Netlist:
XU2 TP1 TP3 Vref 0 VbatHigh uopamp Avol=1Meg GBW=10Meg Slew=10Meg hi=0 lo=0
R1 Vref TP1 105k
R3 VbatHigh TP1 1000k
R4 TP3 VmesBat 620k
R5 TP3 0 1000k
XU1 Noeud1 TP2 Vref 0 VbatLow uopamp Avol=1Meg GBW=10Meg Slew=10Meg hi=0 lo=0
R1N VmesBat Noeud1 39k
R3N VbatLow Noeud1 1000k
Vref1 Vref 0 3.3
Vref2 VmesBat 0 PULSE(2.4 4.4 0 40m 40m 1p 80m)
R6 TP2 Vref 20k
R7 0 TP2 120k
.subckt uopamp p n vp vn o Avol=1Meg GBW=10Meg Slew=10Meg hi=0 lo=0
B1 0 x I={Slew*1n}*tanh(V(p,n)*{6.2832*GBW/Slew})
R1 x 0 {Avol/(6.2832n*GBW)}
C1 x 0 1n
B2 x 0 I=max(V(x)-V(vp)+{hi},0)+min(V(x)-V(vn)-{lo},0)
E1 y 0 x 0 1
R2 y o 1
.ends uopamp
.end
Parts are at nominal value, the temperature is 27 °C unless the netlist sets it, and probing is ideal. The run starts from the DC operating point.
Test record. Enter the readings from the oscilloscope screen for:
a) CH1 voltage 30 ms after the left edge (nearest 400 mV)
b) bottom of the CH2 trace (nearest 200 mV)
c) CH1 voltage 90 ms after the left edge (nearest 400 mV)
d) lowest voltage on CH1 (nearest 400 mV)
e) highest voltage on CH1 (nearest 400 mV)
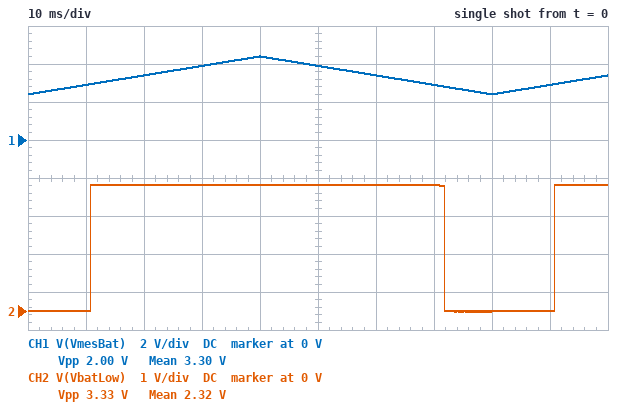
4.0 V
0 V
2.8 V
2.4 V
4.4 V
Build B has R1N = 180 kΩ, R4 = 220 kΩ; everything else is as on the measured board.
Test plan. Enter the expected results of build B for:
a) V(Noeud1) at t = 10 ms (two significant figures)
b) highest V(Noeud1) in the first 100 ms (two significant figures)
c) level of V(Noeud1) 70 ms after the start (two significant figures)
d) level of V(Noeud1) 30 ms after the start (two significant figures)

2.5 V
4.2 V
3.0 V
3.8 V
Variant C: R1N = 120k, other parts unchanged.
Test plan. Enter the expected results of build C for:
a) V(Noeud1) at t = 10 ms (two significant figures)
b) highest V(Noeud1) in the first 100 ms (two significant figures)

2.6 V
4.3 V
